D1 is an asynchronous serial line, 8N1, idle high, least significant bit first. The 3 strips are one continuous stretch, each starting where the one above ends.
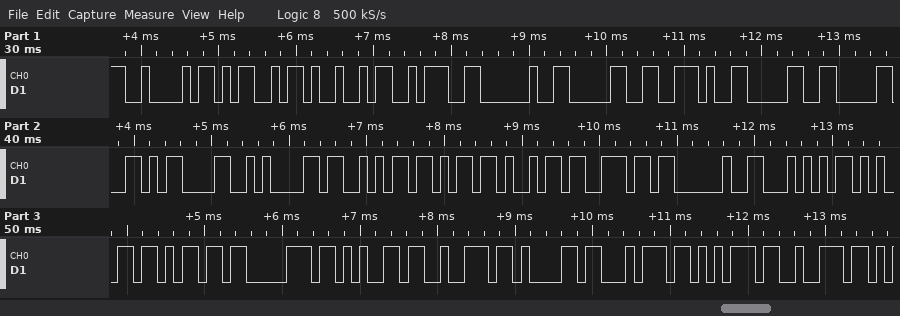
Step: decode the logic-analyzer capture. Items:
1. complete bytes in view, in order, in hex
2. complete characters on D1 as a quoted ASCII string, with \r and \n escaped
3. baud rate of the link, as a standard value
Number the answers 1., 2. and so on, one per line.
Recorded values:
1. 42 4D 49 3A 20 30 2E 30 30 0D 0A 53 6B 69 6E 20 54 65 6D 70 65 72 61 74 75 72
2. "BMI: 0.00\r\nSkin Temperatur"
3. 9600 baud
